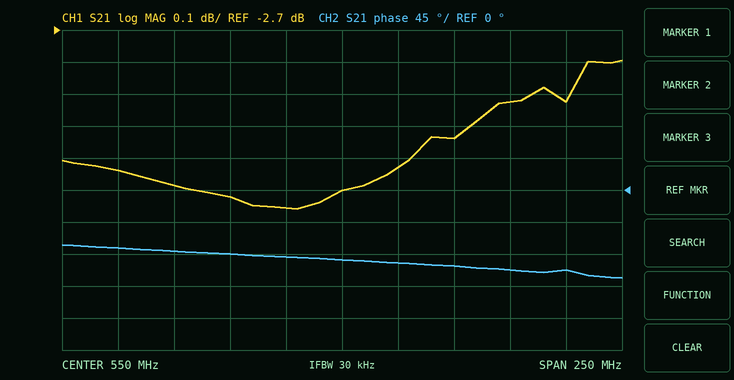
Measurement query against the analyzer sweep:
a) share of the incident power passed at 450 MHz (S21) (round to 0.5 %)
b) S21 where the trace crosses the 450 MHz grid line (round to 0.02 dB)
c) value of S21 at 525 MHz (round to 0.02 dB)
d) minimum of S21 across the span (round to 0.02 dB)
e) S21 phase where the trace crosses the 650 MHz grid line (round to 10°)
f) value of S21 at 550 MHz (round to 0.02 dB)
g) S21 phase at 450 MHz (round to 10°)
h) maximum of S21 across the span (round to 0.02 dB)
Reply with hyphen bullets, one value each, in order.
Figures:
- 48.5 %
- -3.14 dB
- -3.26 dB
- -3.26 dB
- -110°
- -3.20 dB
- -80°
- -2.80 dB
